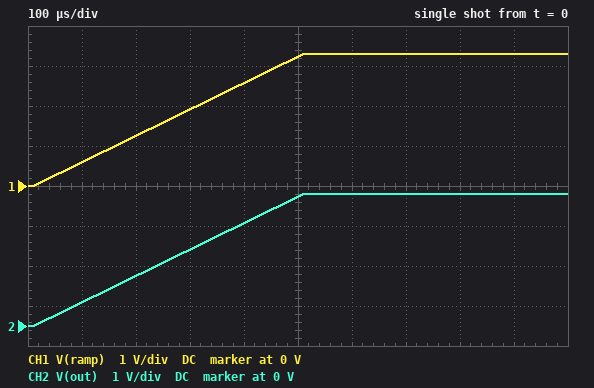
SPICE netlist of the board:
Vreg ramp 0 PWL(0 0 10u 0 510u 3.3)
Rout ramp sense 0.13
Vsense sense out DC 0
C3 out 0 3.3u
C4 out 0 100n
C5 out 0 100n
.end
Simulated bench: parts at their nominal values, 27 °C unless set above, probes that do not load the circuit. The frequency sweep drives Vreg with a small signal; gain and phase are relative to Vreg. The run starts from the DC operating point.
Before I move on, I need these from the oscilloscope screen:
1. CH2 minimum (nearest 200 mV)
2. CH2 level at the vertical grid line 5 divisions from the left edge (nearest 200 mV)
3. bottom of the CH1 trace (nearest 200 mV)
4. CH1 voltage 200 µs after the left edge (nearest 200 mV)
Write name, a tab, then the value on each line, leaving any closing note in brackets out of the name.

CH2 minimum	0 V
CH2 level at the vertical grid line 5 divisions from the left edge	3.2 V
bottom of the CH1 trace	0 V
CH1 voltage 200 µs after the left edge	1.2 V
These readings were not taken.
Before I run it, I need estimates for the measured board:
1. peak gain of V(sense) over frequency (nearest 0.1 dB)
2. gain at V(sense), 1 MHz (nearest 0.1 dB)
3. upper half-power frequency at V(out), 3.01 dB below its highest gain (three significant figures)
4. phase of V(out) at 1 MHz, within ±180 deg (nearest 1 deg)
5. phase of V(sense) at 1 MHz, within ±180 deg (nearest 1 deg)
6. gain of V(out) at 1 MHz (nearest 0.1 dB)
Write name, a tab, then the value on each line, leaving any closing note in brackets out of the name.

peak gain of V(sense) over frequency	0 dB
gain at V(sense), 1 MHz	-9.6 dB
upper half-power frequency at V(out), 3.01 dB below its highest gain	350 kHz
phase of V(out) at 1 MHz, within ±180 deg	-71 deg
phase of V(sense) at 1 MHz, within ±180 deg	-71 deg
gain of V(out) at 1 MHz	-9.6 dB
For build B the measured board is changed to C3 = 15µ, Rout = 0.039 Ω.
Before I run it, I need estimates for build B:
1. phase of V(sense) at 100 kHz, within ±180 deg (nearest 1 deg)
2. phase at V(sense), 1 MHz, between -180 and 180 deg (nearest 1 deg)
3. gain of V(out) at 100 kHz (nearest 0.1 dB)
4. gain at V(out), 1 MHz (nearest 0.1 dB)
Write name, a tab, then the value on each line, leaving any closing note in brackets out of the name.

phase of V(sense) at 100 kHz, within ±180 deg	-20 deg
phase at V(sense), 1 MHz, between -180 and 180 deg	-75 deg
gain of V(out) at 100 kHz	-0.6 dB
gain at V(out), 1 MHz	-11.7 dB
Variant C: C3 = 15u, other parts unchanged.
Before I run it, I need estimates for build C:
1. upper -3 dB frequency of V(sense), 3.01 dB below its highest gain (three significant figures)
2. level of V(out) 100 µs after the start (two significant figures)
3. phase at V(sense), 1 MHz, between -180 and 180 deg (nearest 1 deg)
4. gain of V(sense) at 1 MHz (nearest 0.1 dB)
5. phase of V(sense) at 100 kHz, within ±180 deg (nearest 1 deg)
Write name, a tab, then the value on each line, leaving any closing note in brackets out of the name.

upper -3 dB frequency of V(sense), 3.01 dB below its highest gain	80.5 kHz
level of V(out) 100 µs after the start	580 mV
phase at V(sense), 1 MHz, between -180 and 180 deg	-85 deg
gain of V(sense) at 1 MHz	-21.9 dB
phase of V(sense) at 100 kHz, within ±180 deg	-51 deg
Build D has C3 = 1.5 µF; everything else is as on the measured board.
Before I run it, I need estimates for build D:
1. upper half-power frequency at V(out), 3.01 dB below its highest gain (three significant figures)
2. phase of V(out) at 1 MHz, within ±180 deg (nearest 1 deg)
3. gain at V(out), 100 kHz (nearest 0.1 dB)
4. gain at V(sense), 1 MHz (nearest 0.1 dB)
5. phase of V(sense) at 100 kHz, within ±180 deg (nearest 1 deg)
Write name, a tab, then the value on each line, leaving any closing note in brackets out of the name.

upper half-power frequency at V(out), 3.01 dB below its highest gain	720 kHz
phase of V(out) at 1 MHz, within ±180 deg	-54 deg
gain at V(out), 100 kHz	-0.1 dB
gain at V(sense), 1 MHz	-4.7 dB
phase of V(sense) at 100 kHz, within ±180 deg	-8 deg
